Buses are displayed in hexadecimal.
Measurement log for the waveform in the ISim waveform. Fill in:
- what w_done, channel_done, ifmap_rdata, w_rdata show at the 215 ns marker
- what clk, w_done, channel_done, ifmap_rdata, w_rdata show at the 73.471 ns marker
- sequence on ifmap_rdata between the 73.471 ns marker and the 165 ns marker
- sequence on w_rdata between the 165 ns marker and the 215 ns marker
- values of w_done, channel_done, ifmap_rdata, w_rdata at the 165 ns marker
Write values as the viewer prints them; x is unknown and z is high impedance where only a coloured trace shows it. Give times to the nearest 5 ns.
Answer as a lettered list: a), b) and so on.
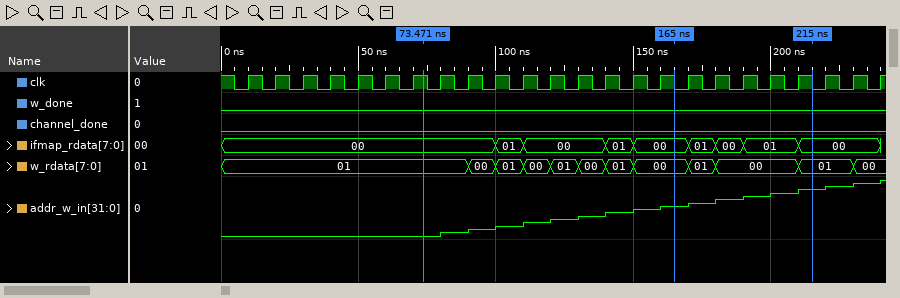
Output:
a) w_done=0, channel_done=0, ifmap_rdata=00, w_rdata=01
b) clk=1, w_done=0, channel_done=0, ifmap_rdata=00, w_rdata=01
c) 00, 01, 00, 01, 00
d) 00, 01, 00, 01
e) w_done=0, channel_done=0, ifmap_rdata=00, w_rdata=00
